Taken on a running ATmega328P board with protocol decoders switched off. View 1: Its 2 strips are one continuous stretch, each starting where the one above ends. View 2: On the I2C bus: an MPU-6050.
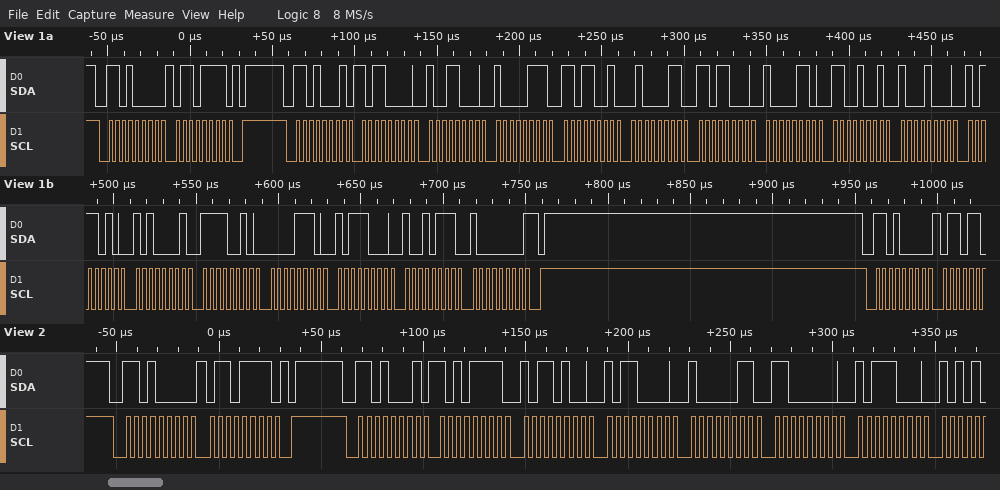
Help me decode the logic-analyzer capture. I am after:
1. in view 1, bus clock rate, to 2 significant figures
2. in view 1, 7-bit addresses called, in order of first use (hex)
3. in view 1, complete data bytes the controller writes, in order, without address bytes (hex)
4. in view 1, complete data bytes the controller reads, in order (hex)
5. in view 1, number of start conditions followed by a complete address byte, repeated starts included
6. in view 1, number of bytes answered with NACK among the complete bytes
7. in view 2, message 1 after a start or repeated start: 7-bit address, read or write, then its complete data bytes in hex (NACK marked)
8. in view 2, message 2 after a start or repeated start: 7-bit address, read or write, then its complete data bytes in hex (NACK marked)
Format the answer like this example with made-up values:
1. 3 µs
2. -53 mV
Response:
1. 250 kHz
2. 0x68
3. 6F
4. B0 98 87 D9 43 D8 86 C9 88 BA A1 F2 0E B8 97 80
5. 3
6. 1
7. 0x68 write: 6F
8. 0x68 read: AF B4 B0 83 C0 B8
